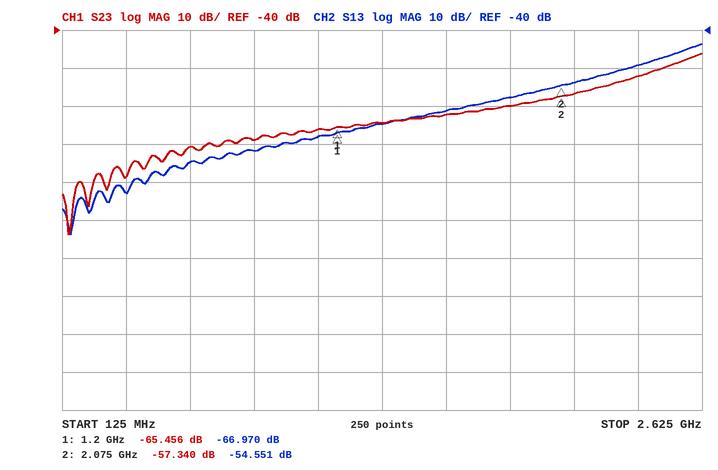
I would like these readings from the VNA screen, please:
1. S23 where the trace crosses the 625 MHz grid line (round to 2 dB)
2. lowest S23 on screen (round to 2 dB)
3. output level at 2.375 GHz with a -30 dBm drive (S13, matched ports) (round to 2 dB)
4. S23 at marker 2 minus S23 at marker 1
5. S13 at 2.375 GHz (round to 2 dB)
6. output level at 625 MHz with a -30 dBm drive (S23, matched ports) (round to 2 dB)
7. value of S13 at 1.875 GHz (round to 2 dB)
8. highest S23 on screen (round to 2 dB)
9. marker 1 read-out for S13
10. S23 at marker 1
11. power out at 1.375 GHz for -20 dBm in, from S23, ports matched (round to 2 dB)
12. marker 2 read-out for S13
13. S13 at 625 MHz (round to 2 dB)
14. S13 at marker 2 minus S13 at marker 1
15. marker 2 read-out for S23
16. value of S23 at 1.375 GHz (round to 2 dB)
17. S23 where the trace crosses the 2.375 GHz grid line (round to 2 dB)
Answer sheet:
-70 dB
-94 dB
-80 dBm
8.116 dB
-50 dB
-100 dBm
-58 dB
-46 dB
-66.970 dB
-65.456 dB
-84 dBm
-54.551 dB
-74 dB
12.419 dB
-57.340 dB
-64 dB
-52 dB
